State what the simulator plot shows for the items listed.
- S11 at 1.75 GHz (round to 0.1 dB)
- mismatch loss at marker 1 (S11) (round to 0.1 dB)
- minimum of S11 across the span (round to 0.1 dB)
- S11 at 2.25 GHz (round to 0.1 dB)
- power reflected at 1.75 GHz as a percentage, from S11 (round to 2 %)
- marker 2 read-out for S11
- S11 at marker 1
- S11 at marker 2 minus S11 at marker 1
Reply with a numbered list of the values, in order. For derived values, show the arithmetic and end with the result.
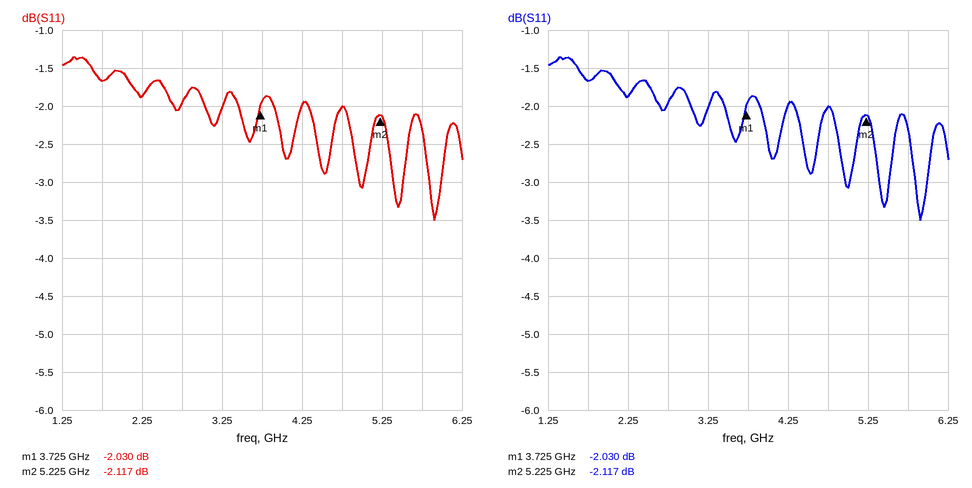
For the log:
1. -1.7 dB
2. −10 log10(1 − 10^(-2.03/10)) ≈ 4.3 dB
3. -3.5 dB
4. -1.9 dB
5. 10^(-1.7/10) ≈ 68 %
6. -2.117 dB
7. -2.030 dB
8. -2.117 − (-2.03) = -0.087 dB
